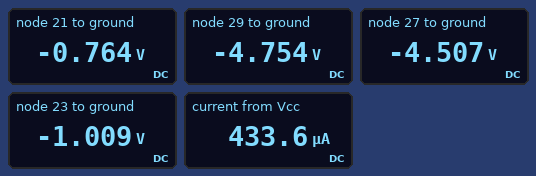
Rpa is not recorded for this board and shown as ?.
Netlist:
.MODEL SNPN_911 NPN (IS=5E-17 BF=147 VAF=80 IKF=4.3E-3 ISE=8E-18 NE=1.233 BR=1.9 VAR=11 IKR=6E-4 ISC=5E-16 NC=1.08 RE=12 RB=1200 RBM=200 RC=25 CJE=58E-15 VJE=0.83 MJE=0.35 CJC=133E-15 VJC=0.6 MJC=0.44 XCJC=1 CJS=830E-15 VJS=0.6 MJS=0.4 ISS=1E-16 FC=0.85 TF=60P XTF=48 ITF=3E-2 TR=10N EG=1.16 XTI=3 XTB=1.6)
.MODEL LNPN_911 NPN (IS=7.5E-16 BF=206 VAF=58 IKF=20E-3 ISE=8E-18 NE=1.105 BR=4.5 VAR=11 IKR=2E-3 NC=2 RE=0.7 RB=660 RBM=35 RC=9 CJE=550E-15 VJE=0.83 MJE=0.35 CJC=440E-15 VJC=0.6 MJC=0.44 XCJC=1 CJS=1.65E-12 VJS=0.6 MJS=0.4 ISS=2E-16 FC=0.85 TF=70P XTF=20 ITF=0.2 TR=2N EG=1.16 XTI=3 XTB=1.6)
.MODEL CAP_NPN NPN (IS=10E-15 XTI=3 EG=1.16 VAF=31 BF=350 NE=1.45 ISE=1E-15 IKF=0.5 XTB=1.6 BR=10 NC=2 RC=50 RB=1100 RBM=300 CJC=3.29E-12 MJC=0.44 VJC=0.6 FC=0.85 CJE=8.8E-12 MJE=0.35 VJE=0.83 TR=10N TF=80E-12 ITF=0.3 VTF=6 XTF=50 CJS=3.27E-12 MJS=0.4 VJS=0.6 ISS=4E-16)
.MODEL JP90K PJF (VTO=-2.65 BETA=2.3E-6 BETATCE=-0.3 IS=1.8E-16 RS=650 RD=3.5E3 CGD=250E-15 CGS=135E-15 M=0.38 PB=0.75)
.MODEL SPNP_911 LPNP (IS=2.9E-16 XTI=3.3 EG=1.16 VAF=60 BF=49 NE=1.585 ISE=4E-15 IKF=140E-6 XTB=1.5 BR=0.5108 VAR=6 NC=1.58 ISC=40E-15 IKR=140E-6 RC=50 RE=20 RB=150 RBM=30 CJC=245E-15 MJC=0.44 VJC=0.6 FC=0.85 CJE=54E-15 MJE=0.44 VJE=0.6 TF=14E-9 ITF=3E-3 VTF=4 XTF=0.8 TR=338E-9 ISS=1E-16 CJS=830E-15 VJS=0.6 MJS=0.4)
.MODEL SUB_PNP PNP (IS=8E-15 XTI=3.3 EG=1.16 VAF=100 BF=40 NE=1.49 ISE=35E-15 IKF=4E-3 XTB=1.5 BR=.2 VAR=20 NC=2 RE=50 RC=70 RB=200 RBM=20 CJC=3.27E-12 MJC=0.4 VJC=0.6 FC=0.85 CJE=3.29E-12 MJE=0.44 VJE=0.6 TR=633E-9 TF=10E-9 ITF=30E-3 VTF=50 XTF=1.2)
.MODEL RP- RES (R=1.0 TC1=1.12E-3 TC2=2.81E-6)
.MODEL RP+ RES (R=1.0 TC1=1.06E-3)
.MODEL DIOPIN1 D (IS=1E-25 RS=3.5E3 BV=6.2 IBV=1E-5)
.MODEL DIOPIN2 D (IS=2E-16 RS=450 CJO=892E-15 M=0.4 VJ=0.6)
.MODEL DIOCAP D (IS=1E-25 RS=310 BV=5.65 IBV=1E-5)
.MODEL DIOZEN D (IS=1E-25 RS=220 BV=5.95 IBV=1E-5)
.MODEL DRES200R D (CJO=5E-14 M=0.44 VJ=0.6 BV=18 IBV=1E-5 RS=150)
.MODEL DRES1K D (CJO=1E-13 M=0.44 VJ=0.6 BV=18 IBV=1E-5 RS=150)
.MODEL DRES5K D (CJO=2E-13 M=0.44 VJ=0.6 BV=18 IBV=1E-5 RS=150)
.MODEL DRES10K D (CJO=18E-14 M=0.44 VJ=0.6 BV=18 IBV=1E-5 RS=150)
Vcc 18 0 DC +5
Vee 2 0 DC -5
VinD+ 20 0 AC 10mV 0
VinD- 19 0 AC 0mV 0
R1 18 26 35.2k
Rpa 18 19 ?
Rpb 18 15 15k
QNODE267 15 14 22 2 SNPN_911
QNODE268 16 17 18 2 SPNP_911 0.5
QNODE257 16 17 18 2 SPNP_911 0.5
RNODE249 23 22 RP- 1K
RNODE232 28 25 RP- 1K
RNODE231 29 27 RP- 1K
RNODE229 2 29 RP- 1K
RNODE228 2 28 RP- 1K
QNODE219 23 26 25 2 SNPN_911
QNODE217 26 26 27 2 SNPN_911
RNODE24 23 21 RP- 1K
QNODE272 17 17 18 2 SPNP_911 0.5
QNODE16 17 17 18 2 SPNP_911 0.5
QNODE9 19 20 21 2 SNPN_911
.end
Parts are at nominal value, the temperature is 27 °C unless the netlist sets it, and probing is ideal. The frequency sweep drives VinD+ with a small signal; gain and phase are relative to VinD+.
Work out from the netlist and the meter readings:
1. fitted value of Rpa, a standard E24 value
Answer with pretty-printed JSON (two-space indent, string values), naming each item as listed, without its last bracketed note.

{
  "fitted value of Rpa, a standard E24 value": "27 kΩ"
}
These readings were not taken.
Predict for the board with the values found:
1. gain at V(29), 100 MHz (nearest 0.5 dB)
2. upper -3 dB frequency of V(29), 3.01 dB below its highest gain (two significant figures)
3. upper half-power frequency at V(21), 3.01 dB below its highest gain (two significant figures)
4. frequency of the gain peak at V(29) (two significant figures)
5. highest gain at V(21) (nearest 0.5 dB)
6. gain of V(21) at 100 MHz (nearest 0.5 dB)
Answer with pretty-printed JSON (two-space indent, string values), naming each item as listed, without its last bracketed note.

{
  "gain at V(29), 100 MHz": "-31.5 dB",
  "upper -3 dB frequency of V(29), 3.01 dB below its highest gain": "410 MHz",
  "upper half-power frequency at V(21), 3.01 dB below its highest gain": "650 MHz",
  "frequency of the gain peak at V(29)": "180 MHz",
  "highest gain at V(21)": "0 dB",
  "gain of V(21) at 100 MHz": "0 dB"
}
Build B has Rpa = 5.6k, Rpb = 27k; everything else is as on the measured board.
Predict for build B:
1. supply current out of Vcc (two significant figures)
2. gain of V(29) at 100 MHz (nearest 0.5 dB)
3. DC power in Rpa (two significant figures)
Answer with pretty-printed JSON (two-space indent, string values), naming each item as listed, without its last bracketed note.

{
  "supply current out of Vcc": "1.1 mA",
  "gain of V(29) at 100 MHz": "-31.5 dB",
  "DC power in Rpa": "4.5 mW"
}
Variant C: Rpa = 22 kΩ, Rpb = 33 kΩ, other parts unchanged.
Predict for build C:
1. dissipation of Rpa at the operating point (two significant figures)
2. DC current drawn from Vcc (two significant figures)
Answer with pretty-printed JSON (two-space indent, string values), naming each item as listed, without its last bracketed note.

{
  "dissipation of Rpa at the operating point": "1.1 mW",
  "DC current drawn from Vcc": "480 µA"
}
